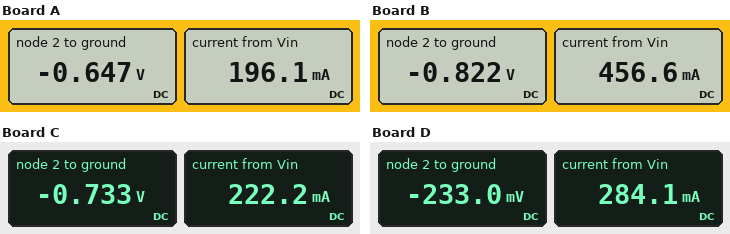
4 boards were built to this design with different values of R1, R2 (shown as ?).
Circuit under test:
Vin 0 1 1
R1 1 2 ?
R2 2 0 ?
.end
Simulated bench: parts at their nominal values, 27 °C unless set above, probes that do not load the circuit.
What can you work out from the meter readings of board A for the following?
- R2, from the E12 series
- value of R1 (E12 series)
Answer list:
3.3 Ω
1.8 Ω
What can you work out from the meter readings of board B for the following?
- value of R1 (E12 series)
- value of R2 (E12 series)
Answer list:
0.39 Ω
1.8 Ω
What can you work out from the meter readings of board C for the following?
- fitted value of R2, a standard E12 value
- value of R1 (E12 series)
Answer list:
3.3 Ω
1.2 Ω
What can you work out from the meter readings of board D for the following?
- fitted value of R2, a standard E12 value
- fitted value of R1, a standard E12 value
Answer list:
0.82 Ω
2.7 Ω
